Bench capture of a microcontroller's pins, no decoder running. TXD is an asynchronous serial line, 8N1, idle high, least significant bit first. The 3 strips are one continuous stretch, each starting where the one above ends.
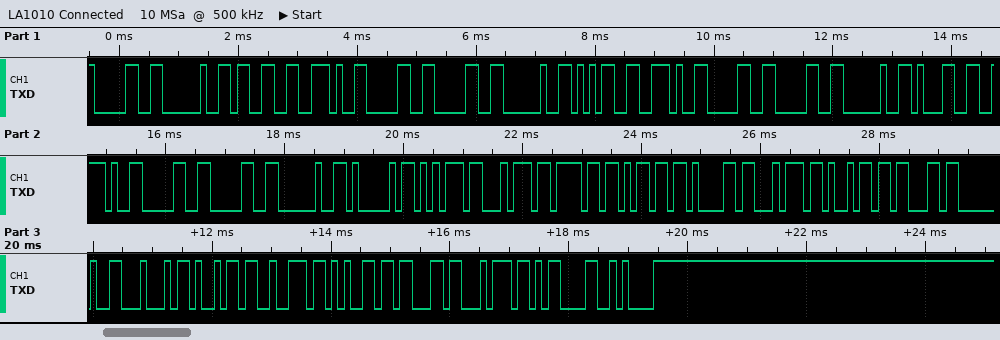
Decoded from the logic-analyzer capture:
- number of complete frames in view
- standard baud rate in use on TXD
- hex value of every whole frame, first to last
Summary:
35
9600 baud
0x30 0x20 0x33 0x2E 0x30 0x30 0x20 0x35 0x2E 0x30 0x30 0x20 0x31 0x2E 0x30 0x30 0x20 0x41 0x75 0x74 0x6F 0x6D 0x61 0x74 0x69 0x63 0x20 0x44 0x69 0x72 0x65 0x63 0x74 0x0D 0x0A
